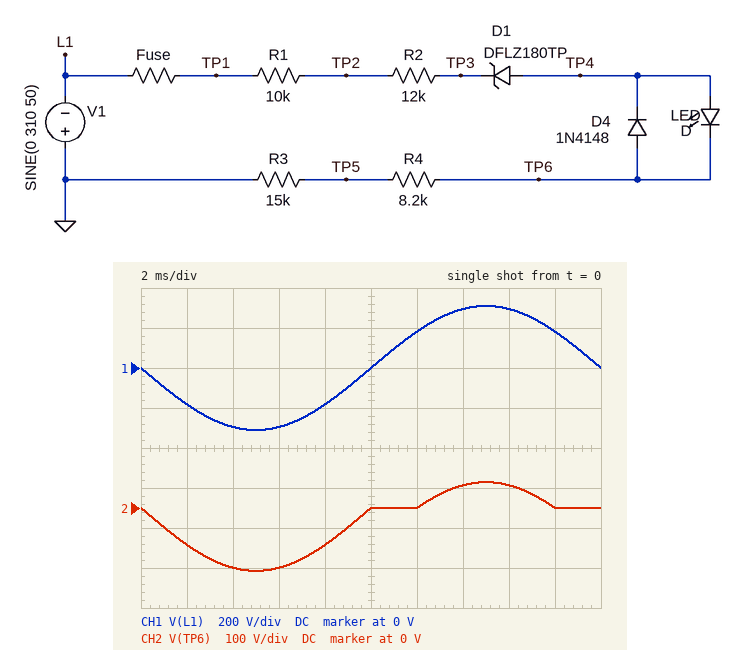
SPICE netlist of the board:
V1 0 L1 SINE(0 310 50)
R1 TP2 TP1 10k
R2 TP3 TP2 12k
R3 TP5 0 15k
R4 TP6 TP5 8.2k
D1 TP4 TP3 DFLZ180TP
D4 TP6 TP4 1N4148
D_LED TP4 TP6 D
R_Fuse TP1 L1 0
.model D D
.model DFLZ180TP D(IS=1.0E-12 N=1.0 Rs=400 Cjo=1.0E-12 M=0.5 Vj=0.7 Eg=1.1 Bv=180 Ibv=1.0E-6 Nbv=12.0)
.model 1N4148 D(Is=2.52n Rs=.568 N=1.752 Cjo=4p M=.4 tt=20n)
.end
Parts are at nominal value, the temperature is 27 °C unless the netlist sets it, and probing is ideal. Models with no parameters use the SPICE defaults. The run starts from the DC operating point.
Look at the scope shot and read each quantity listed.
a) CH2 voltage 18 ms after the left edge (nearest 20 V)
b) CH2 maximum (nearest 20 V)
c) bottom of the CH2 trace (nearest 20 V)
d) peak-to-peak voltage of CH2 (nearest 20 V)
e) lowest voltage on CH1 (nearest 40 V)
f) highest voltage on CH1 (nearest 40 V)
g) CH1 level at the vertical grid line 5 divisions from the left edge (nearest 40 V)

0 V
60 V
-160 V
220 V
-320 V
320 V
0 V
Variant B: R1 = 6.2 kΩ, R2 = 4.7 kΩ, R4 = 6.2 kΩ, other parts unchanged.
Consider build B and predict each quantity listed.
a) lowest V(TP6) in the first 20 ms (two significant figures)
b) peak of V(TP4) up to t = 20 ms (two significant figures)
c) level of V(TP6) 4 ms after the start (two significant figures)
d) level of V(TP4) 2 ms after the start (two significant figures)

-200 V
83 V
-190 V
-120 V
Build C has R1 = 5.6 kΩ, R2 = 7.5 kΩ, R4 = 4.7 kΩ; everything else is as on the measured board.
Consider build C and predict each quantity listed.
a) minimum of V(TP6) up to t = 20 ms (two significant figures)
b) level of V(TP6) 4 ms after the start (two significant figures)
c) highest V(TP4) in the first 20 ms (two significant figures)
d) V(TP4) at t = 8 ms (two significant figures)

-180 V
-170 V
76 V
-110 V
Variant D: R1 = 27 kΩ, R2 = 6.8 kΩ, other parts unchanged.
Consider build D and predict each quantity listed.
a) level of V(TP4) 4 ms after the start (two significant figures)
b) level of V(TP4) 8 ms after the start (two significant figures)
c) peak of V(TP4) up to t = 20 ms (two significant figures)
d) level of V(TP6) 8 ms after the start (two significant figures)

-120 V
-74 V
52 V
-73 V
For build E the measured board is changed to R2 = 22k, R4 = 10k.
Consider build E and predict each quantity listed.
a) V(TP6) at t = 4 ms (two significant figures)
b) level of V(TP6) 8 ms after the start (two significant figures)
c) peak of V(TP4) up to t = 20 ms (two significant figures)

-130 V
-79 V
56 V
